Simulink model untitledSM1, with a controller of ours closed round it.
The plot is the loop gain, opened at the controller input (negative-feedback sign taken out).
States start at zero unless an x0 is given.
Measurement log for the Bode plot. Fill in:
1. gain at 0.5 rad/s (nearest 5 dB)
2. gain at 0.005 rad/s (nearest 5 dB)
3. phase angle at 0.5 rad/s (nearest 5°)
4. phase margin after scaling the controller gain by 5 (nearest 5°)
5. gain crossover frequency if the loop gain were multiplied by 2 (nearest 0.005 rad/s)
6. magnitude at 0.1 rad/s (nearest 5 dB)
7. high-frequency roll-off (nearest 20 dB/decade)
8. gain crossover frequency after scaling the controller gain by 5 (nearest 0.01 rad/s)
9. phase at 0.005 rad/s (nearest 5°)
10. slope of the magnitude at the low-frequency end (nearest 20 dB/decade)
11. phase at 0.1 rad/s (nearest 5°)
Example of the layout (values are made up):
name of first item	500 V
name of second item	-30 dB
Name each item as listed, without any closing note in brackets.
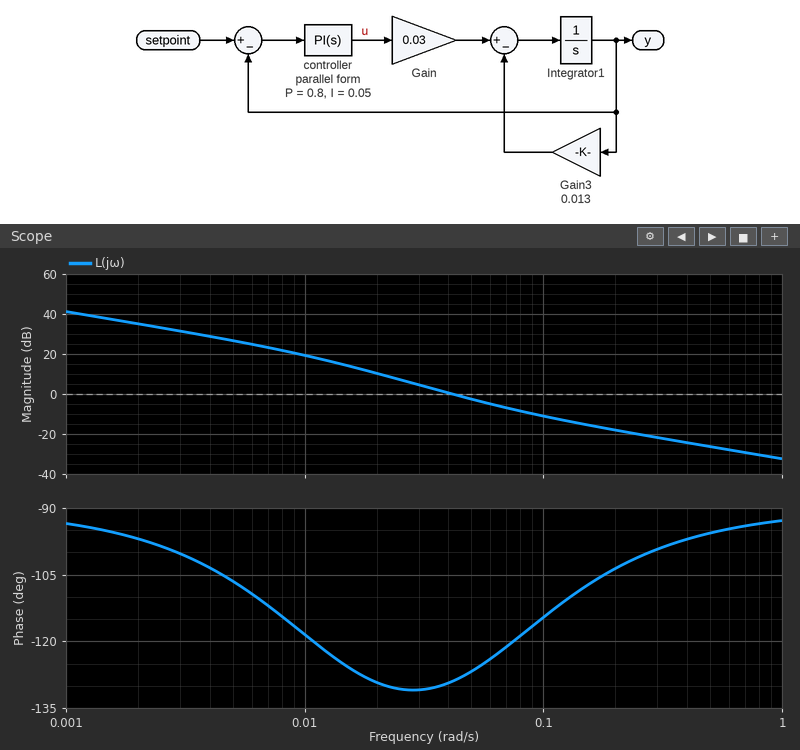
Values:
gain at 0.5 rad/s	-25 dB
gain at 0.005 rad/s	25 dB
phase angle at 0.5 rad/s	-95°
phase margin after scaling the controller gain by 5	70°
gain crossover frequency if the loop gain were multiplied by 2	0.065 rad/s
magnitude at 0.1 rad/s	-10 dB
high-frequency roll-off	-20 dB/decade
gain crossover frequency after scaling the controller gain by 5	0.13 rad/s
phase at 0.005 rad/s	-105°
slope of the magnitude at the low-frequency end	-20 dB/decade
phase at 0.1 rad/s	-115°
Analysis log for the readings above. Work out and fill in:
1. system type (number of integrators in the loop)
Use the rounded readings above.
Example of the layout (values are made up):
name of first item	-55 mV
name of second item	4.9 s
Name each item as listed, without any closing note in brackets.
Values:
system type	1
